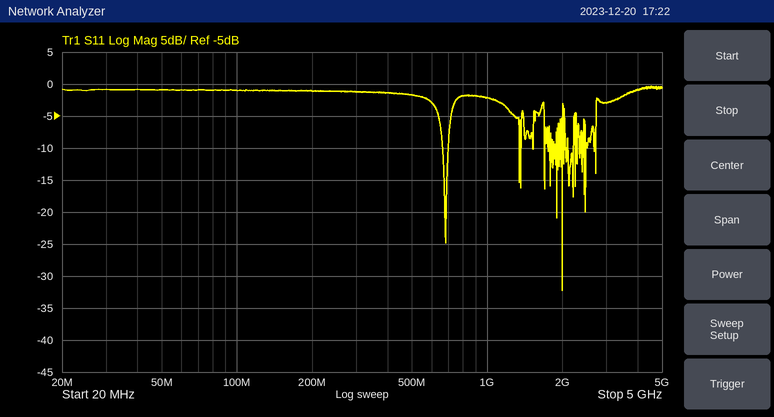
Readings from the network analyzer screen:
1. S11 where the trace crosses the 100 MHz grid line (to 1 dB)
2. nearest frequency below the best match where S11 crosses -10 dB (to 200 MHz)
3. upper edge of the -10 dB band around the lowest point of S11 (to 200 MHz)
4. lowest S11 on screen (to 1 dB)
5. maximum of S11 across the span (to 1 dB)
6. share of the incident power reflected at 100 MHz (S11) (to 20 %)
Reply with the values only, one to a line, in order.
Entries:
-1 dB
2.0 GHz
2.0 GHz
-32 dB
0 dB
80 %
